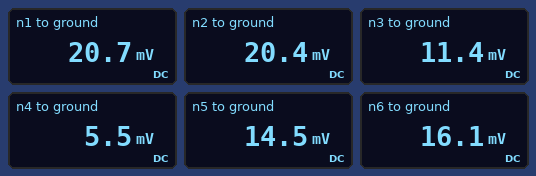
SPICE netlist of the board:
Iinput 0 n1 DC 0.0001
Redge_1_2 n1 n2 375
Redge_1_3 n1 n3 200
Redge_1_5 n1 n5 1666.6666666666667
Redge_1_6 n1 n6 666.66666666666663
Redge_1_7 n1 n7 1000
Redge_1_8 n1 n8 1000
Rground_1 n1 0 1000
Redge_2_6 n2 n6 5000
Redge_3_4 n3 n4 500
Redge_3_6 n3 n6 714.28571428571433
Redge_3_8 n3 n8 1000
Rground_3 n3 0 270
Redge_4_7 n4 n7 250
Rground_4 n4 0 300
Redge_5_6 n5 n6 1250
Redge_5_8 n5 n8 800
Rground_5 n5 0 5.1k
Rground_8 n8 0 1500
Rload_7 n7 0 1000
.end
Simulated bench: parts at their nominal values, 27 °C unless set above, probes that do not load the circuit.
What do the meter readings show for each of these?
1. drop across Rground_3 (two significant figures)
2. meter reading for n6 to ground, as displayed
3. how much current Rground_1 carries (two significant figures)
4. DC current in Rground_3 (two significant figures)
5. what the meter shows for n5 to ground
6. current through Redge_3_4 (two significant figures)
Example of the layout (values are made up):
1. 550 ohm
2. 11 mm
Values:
1. 11 mV
2. 16.1 mV
3. 21 µA
4. 42 µA
5. 14.5 mV
6. 12 µA
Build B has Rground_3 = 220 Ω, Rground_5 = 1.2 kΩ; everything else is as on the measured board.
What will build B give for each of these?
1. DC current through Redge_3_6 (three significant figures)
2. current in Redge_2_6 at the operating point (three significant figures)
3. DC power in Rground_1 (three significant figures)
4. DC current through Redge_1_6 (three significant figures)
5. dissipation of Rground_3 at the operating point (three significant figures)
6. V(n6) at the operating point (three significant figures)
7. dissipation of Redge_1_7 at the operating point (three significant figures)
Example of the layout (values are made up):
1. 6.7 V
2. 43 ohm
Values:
1. 5.81 µA
2. 955 nA
3. 355 nW
4. 7.70 µA
5. 416 nW
6. 13.7 mV
7. 157 nW
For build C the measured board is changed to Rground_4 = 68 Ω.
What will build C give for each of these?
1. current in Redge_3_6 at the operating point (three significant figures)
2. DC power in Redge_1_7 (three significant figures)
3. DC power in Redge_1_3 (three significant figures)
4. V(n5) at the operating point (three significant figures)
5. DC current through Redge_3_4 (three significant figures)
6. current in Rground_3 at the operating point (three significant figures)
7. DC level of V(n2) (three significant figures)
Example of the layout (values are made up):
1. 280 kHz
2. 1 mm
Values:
1. 6.60 µA
2. 227 nW
3. 432 nW
4. 13.6 mV
5. 16.8 µA
6. 38.0 µA
7. 19.2 mV
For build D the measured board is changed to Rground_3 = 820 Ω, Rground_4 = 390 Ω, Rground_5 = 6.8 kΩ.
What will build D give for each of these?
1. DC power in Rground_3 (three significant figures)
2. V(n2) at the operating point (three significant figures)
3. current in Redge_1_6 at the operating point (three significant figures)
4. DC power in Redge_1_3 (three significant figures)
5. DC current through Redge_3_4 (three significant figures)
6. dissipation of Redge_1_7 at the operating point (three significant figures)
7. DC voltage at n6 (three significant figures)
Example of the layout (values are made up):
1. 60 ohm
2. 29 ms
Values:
1. 442 nW
2. 26.4 mV
3. 6.10 µA
4. 292 nW
5. 19.1 µA
6. 253 nW
7. 22.6 mV
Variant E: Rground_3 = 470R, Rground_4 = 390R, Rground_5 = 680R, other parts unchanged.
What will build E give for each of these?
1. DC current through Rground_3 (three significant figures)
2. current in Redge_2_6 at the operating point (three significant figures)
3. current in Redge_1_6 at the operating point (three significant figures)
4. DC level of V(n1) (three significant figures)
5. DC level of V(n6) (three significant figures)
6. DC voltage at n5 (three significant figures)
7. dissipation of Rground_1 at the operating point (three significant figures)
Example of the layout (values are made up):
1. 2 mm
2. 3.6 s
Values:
1. 29.0 µA
2. 978 nA
3. 7.89 µA
4. 21.6 mV
5. 16.4 mV
6. 10.0 mV
7. 467 nW
